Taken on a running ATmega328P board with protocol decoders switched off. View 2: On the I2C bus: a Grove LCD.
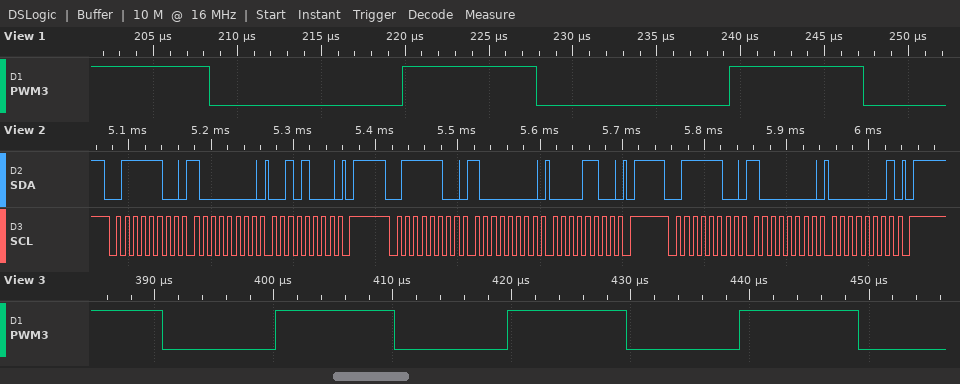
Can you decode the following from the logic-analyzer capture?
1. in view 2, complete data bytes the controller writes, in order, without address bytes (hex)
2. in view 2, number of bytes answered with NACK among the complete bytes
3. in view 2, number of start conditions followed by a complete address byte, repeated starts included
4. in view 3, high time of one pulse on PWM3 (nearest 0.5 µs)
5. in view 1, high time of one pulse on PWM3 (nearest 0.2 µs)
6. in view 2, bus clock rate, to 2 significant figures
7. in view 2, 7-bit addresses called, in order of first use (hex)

80 28 80 0C 80 01
0
3
10.0 µs
8.0 µs
100 kHz
0x3E
